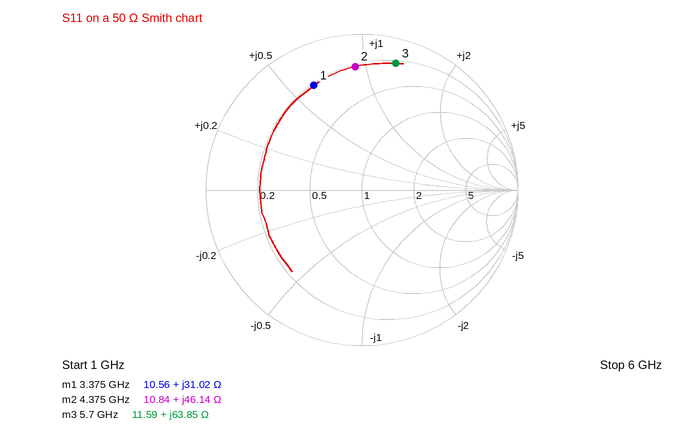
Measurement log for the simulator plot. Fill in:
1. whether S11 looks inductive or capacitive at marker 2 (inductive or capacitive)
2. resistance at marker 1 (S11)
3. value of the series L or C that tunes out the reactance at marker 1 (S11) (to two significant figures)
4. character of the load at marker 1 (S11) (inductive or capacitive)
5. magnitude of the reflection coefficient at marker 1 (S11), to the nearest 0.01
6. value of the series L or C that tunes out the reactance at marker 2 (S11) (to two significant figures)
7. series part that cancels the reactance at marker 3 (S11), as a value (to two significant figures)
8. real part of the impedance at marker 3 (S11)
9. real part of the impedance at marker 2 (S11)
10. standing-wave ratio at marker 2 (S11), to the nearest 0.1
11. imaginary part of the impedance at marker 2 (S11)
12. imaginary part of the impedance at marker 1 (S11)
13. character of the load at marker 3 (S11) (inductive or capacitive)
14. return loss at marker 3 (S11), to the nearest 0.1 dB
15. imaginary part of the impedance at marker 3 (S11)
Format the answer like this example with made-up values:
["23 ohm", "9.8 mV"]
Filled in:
["inductive", "10.56 Ω", "1.5 pF", "inductive", "0.74", "790 fF", "440 fF", "11.59 Ω", "10.84 Ω", "8.6", "+46.14 Ω", "+31.02 Ω", "inductive", "1.5 dB", "+63.85 Ω"]
